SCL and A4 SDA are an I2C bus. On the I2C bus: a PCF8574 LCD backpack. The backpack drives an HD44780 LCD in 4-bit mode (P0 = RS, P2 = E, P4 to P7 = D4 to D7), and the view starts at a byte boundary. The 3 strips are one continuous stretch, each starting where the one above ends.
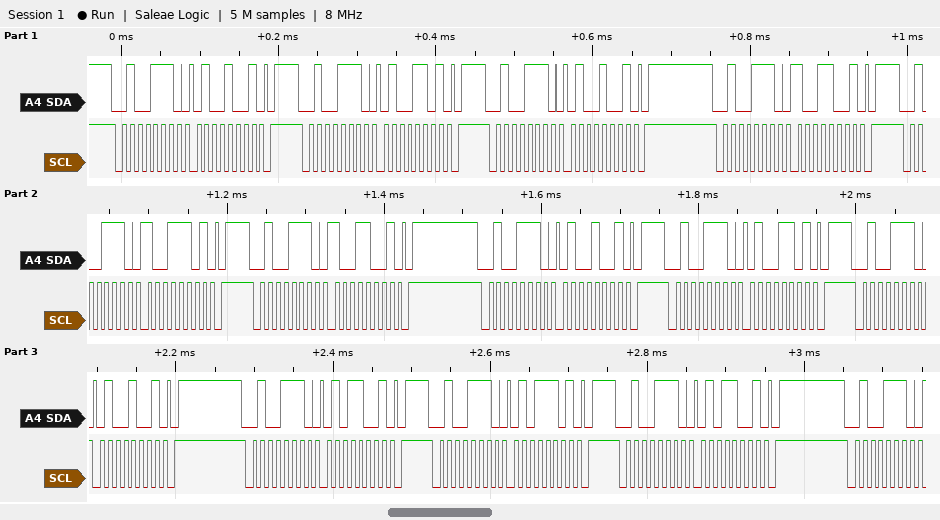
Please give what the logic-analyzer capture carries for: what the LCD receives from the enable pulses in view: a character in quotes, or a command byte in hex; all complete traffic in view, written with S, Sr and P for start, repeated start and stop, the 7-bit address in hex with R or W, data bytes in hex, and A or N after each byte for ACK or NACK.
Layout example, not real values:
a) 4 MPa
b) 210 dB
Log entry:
a) 'I' 'E'
b) S 27W A 49 A P S 27W A 4D A P S 27W A 49 A P S 27W A 99 A P S 27W A 9D A P S 27W A 99 A P S 27W A 49 A P S 27W A 4D A P S 27W A 49 A P S 27W A 59 A P S 27W A 5D A P S 27W A 59 A P S 27W A
